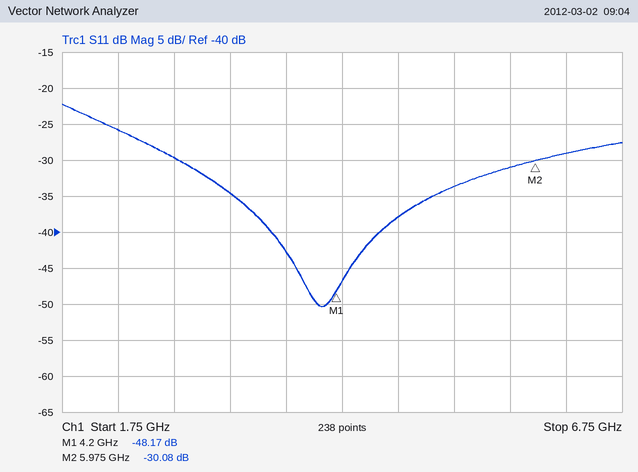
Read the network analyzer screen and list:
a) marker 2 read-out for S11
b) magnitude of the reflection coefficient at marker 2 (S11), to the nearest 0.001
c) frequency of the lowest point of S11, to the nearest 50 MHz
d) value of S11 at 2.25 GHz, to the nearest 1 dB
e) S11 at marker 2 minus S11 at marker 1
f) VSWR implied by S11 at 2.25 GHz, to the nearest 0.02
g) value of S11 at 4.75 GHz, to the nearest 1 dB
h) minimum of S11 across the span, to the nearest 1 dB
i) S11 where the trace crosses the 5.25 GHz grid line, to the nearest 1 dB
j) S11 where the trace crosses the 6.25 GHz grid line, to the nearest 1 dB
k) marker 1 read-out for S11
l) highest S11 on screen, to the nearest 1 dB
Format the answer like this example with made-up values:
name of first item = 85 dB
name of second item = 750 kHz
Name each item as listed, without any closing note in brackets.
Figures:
marker 2 read-out for S11 = -30.08 dB
magnitude of the reflection coefficient at marker 2 (S11), to the nearest 0.001 = 0.031
frequency of the lowest point of S11, to the nearest 50 MHz = 4.05 GHz
value of S11 at 2.25 GHz, to the nearest 1 dB = -26 dB
S11 at marker 2 minus S11 at marker 1 = 18.09 dB
VSWR implied by S11 at 2.25 GHz, to the nearest 0.02 = 1.10
value of S11 at 4.75 GHz, to the nearest 1 dB = -38 dB
minimum of S11 across the span, to the nearest 1 dB = -50 dB
S11 where the trace crosses the 5.25 GHz grid line, to the nearest 1 dB = -34 dB
S11 where the trace crosses the 6.25 GHz grid line, to the nearest 1 dB = -29 dB
marker 1 read-out for S11 = -48.17 dB
highest S11 on screen, to the nearest 1 dB = -22 dB
